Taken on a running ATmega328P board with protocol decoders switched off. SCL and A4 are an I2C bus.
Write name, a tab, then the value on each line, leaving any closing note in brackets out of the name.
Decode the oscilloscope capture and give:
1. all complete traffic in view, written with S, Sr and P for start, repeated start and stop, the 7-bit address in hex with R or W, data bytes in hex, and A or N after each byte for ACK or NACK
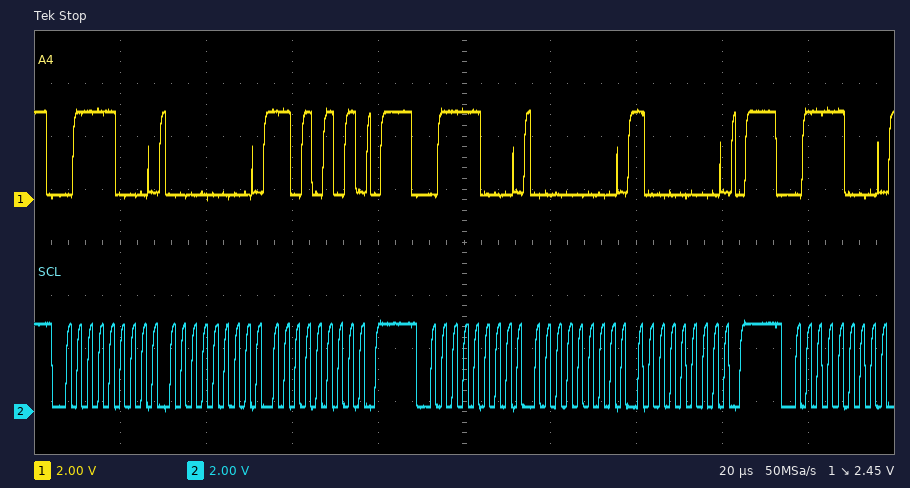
all complete traffic in view, written with S, Sr and P for start, repeated start and stop, the 7-bit address in hex with R or W, data bytes in hex, and A or N after each byte for ACK or NACK	S 3CW A 00 A D5 A P S 3CW A 00 A 80 A P S 3CW A
